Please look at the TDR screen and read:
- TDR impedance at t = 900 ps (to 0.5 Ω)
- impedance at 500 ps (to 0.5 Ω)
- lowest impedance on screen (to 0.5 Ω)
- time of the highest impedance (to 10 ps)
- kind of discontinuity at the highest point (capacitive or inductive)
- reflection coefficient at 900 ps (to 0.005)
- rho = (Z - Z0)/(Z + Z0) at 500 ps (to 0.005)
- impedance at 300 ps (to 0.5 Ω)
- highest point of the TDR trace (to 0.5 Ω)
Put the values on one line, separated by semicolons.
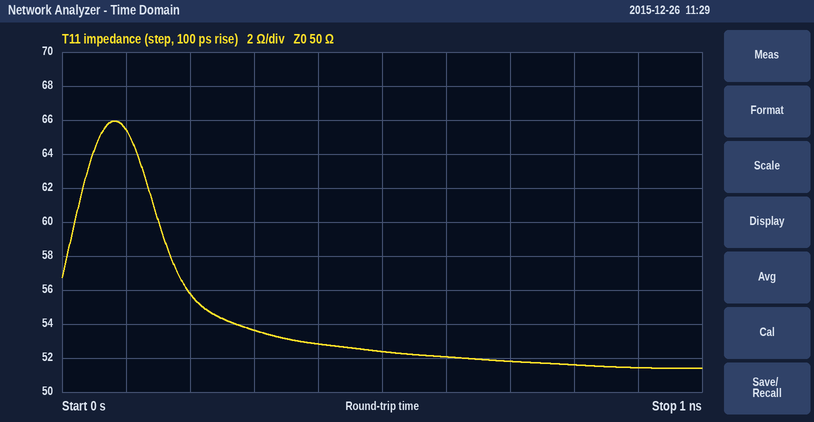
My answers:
51.5 Ω; 52.5 Ω; 51.5 Ω; 80 ps; inductive; +0.015; +0.025; 53.5 Ω; 66.0 Ω
